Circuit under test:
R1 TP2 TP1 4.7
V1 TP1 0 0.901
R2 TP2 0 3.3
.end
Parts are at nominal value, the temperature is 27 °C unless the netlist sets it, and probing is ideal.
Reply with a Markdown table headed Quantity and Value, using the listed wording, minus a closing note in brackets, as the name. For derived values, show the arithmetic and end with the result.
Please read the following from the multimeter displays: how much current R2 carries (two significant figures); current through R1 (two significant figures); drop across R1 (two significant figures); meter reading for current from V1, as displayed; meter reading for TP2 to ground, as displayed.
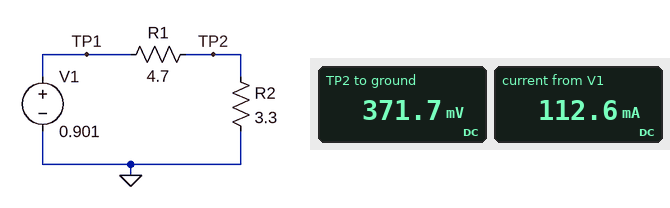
| Quantity | Value |
|---|---|
| how much current R2 carries | (371.7 mV) / 3.3 Ω = 110 mA |
| current through R1 | (901 mV - 371.7 mV) / 4.7 Ω = 110 mA |
| drop across R1 | 901 mV - 371.7 mV = 530 mV |
| meter reading for current from V1, as displayed | 112.6 mA |
| meter reading for TP2 to ground, as displayed | 371.7 mV |
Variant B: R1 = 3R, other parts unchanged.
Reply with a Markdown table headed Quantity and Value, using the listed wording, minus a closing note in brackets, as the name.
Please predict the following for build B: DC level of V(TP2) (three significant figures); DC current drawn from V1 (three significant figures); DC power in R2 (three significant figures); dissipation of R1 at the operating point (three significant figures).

| Quantity | Value |
|---|---|
| DC level of V(TP2) | 472 mV |
| DC current drawn from V1 | 143 mA |
| DC power in R2 | 67.5 mW |
| dissipation of R1 at the operating point | 61.4 mW |
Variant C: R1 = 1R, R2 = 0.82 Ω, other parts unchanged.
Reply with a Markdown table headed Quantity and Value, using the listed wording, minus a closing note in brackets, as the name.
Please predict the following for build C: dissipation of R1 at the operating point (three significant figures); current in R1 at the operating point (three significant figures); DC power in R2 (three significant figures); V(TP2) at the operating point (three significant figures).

| Quantity | Value |
|---|---|
| dissipation of R1 at the operating point | 245 mW |
| current in R1 at the operating point | 495 mA |
| DC power in R2 | 201 mW |
| V(TP2) at the operating point | 406 mV |
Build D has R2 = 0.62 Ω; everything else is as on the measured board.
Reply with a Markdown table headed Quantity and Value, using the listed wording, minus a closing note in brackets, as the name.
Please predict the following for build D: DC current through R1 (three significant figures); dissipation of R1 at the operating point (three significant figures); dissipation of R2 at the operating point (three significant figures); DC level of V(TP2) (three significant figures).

| Quantity | Value |
|---|---|
| DC current through R1 | 169 mA |
| dissipation of R1 at the operating point | 135 mW |
| dissipation of R2 at the operating point | 17.8 mW |
| DC level of V(TP2) | 105 mV |
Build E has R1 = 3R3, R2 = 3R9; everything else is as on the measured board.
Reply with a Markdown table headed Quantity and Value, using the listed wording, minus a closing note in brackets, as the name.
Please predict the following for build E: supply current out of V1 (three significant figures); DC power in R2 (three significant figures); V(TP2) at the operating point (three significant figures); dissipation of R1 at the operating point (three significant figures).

| Quantity | Value |
|---|---|
| supply current out of V1 | 125 mA |
| DC power in R2 | 61.1 mW |
| V(TP2) at the operating point | 488 mV |
| dissipation of R1 at the operating point | 51.7 mW |
